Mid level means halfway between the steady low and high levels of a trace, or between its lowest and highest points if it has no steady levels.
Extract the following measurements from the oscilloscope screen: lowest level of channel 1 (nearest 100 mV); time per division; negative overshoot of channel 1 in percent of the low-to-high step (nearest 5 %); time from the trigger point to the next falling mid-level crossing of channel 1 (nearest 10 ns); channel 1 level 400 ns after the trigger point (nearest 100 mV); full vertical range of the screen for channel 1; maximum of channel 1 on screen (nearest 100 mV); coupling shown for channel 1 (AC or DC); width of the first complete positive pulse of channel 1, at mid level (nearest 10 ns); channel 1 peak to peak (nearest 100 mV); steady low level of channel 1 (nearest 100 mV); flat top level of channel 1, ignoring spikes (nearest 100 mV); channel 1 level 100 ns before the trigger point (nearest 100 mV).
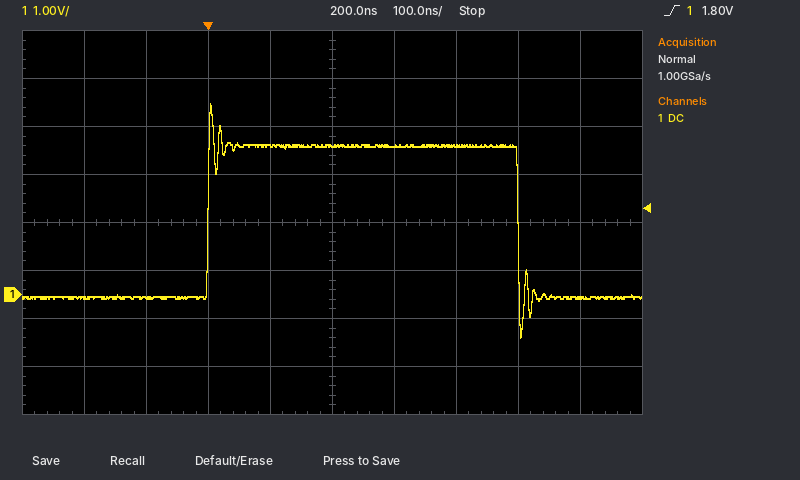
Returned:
-900 mV
100 ns
25 %
500 ns
3.1 V
8 V
4.0 V
DC
500 ns
4.9 V
-100 mV
3.1 V
-100 mV
